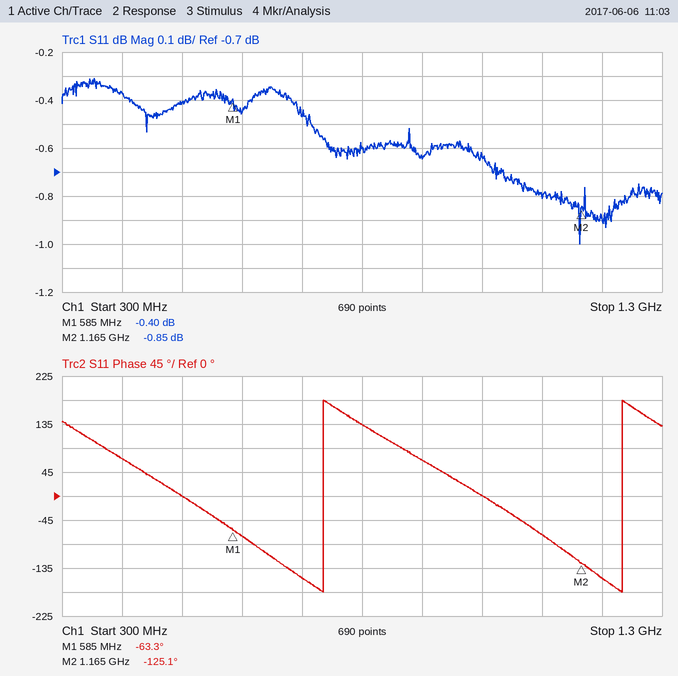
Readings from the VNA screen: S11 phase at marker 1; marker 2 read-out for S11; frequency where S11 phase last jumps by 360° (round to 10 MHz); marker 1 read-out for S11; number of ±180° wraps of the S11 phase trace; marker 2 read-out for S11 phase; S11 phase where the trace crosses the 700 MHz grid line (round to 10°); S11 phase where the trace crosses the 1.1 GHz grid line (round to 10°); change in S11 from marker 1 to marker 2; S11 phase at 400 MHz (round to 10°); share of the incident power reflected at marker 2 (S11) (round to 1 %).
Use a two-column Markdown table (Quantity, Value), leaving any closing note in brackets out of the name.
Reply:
| Quantity | Value |
|---|---|
| S11 phase at marker 1 | -63.3° |
| marker 2 read-out for S11 | -0.85 dB |
| frequency where S11 phase last jumps by 360° | 1.23 GHz |
| marker 1 read-out for S11 | -0.40 dB |
| number of ±180° wraps of the S11 phase trace | 2 |
| marker 2 read-out for S11 phase | -125.1° |
| S11 phase where the trace crosses the 700 MHz grid line | -150° |
| S11 phase where the trace crosses the 1.1 GHz grid line | -70° |
| change in S11 from marker 1 to marker 2 | -0.45 dB |
| S11 phase at 400 MHz | 70° |
| share of the incident power reflected at marker 2 (S11) | 82 % |
